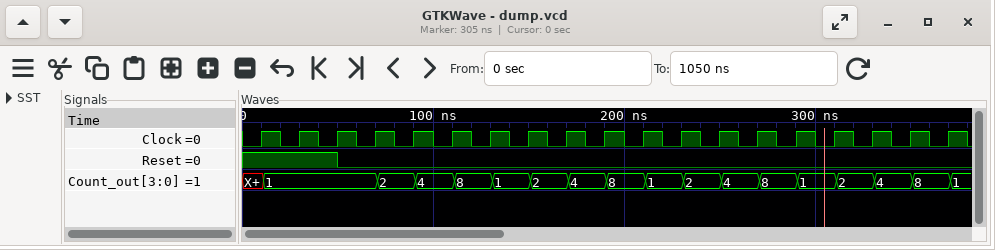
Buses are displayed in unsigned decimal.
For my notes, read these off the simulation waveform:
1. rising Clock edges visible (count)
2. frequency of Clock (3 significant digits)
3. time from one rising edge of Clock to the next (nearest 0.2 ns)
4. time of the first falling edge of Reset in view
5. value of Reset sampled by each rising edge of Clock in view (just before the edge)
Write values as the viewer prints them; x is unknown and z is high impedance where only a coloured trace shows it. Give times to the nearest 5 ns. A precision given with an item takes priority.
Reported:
19
50.0 MHz
20 ns
50 ns
1 1 1 0 0 0 0 0 0 0 0 0 0 0 0 0 0 0 0
